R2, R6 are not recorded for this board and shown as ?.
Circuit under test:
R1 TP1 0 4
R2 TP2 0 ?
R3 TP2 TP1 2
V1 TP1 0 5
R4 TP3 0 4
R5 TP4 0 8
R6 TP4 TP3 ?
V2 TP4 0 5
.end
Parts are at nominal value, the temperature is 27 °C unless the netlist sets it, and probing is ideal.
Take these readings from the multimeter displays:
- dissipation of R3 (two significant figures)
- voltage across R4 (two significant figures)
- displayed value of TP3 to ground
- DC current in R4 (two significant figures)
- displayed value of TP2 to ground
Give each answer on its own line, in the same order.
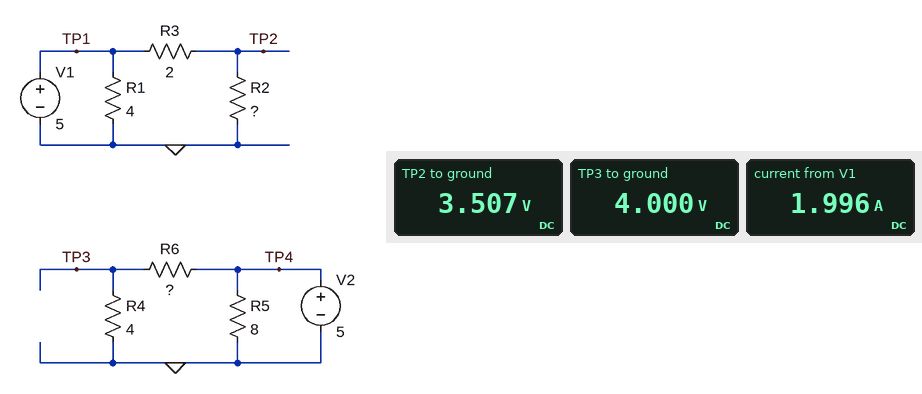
1.1 W
4.0 V
4.000 V
1.0 A
3.507 V
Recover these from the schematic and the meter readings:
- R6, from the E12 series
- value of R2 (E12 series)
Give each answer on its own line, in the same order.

1 Ω
4.7 Ω
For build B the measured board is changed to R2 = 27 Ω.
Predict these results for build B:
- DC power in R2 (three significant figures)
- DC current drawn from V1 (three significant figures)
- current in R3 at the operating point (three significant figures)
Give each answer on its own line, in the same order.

803 mW
1.42 A
172 mA
